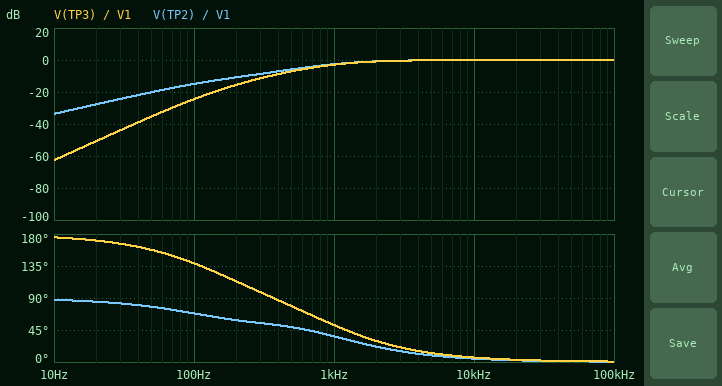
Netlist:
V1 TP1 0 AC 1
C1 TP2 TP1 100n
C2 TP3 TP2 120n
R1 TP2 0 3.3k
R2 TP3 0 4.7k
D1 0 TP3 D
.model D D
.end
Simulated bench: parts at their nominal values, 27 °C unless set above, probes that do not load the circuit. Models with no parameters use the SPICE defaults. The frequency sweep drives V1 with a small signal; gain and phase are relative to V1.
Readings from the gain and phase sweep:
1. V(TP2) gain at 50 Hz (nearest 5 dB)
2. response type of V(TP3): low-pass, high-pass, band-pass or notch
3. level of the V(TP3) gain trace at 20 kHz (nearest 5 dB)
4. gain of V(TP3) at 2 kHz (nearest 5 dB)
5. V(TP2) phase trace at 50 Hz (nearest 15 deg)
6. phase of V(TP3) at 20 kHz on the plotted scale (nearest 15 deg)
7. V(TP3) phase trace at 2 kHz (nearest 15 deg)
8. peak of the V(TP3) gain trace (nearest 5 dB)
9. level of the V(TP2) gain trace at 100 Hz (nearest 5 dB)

-20 dB
high-pass
0 dB
0 dB
75 deg
0 deg
30 deg
0 dB
-15 dB
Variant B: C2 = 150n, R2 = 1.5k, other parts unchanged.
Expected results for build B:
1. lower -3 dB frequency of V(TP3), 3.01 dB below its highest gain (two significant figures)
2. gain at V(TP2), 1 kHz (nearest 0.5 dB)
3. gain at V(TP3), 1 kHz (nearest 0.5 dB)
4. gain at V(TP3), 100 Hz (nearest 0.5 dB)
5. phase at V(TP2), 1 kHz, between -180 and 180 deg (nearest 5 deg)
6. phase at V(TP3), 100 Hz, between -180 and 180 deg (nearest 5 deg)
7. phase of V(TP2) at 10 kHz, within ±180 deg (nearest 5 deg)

2.1 kHz
-5.5 dB
-7.5 dB
-32.0 dB
40 deg
145 deg
10 deg
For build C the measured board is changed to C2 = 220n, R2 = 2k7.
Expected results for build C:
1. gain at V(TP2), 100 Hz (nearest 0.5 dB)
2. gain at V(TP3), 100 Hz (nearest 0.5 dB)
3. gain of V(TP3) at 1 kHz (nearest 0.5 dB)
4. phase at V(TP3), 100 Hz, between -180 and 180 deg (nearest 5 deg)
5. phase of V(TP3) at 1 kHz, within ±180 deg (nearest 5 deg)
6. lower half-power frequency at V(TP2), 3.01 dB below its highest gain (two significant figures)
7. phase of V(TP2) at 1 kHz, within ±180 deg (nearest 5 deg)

-16.0 dB
-25.0 dB
-4.0 dB
130 deg
55 deg
1.2 kHz
40 deg
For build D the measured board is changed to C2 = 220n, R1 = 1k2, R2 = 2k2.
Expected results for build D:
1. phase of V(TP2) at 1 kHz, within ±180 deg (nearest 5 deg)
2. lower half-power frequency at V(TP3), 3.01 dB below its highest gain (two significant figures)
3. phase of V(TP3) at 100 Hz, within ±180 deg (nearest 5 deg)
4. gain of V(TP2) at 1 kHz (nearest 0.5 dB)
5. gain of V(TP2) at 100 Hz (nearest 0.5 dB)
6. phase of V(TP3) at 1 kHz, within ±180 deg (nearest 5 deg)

60 deg
2.2 kHz
150 deg
-7.5 dB
-23.0 dB
75 deg
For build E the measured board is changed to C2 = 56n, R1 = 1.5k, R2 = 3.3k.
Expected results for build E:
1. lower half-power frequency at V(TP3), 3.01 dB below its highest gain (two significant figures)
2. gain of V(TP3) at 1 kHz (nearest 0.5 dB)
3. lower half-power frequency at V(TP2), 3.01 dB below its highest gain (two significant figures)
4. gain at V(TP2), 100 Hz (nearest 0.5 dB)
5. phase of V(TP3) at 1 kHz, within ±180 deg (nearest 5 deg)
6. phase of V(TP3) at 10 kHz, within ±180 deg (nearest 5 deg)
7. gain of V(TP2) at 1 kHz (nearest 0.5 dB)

2.0 kHz
-7.5 dB
1.7 kHz
-20.5 dB
90 deg
15 deg
-5.0 dB
